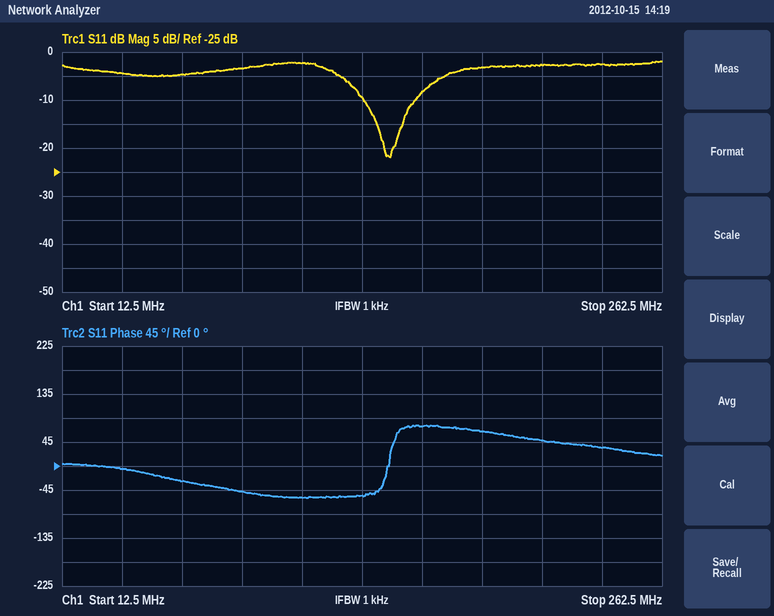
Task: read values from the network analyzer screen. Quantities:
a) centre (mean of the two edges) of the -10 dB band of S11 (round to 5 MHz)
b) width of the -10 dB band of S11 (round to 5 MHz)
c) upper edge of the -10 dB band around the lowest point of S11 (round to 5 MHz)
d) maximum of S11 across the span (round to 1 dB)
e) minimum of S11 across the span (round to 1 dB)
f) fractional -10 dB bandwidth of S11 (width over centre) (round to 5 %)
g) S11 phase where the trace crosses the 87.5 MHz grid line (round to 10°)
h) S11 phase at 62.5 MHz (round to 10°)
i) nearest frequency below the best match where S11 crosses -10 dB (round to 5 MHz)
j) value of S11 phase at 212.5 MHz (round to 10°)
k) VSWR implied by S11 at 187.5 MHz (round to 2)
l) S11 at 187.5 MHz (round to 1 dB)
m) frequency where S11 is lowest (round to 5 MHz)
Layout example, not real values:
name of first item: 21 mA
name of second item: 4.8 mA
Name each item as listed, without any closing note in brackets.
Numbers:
centre (mean of the two edges) of the -10 dB band of S11: 150 MHz
width of the -10 dB band of S11: 20 MHz
upper edge of the -10 dB band around the lowest point of S11: 160 MHz
maximum of S11 across the span: -2 dB
minimum of S11 across the span: -22 dB
fractional -10 dB bandwidth of S11 (width over centre): 15 %
S11 phase where the trace crosses the 87.5 MHz grid line: -50°
S11 phase at 62.5 MHz: -30°
nearest frequency below the best match where S11 crosses -10 dB: 140 MHz
value of S11 phase at 212.5 MHz: 50°
VSWR implied by S11 at 187.5 MHz: 6
S11 at 187.5 MHz: -3 dB
frequency where S11 is lowest: 150 MHz
